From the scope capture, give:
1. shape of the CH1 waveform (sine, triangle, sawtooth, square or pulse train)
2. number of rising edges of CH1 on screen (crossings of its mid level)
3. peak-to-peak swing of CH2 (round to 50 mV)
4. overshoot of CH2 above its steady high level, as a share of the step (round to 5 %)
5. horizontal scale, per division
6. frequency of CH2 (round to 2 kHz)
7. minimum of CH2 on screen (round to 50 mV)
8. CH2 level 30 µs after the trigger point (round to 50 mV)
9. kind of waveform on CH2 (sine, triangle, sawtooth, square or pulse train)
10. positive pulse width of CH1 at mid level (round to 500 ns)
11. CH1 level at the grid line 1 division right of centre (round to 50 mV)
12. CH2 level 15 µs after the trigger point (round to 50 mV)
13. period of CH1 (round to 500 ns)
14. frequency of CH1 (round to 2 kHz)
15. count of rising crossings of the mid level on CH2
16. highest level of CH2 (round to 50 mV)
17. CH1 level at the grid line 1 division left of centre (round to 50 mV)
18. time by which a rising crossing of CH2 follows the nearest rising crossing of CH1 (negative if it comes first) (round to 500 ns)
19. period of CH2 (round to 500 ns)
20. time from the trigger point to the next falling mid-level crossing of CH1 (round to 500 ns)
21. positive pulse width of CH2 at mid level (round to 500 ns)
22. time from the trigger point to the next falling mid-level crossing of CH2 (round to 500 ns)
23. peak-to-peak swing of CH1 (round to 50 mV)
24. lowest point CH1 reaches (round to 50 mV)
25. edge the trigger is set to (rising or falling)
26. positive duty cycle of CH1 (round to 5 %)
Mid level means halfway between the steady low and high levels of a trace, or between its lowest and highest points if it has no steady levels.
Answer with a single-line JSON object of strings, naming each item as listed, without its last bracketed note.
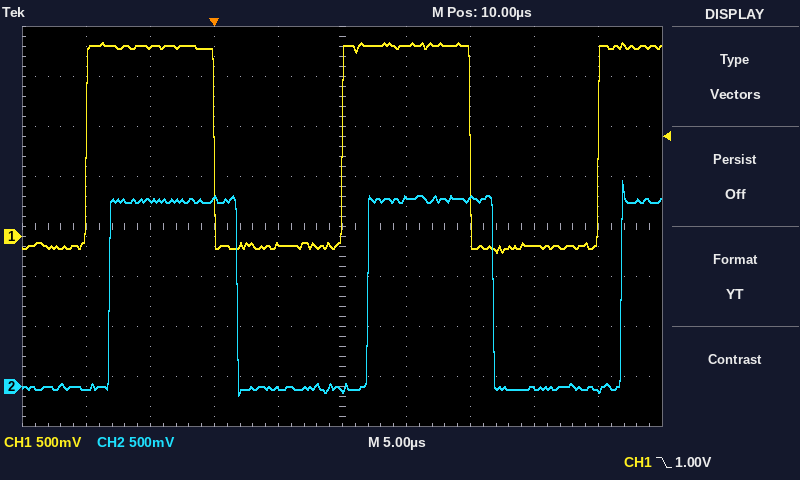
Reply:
{"shape of the CH1 waveform": "square", "number of rising edges of CH1 on screen": "3", "peak-to-peak swing of CH2": "2.15 V", "overshoot of CH2 above its steady high level, as a share of the step": "10 %", "horizontal scale, per division": "5 µs", "frequency of CH2": "50 kHz", "minimum of CH2 on screen": "-100 mV", "CH2 level 30 µs after the trigger point": "-50 mV", "kind of waveform on CH2": "square", "positive pulse width of CH1 at mid level": "10.0 µs", "CH1 level at the grid line 1 division right of centre": "1.90 V", "CH2 level 15 µs after the trigger point": "1.90 V", "period of CH1": "20.0 µs", "frequency of CH1": "50 kHz", "count of rising crossings of the mid level on CH2": "3", "highest level of CH2": "2.05 V", "CH1 level at the grid line 1 division left of centre": "-100 mV", "time by which a rising crossing of CH2 follows the nearest rising crossing of CH1 (negative if it comes first)": "+2.0 µs", "period of CH2": "20.0 µs", "time from the trigger point to the next falling mid-level crossing of CH1": "20.0 µs", "positive pulse width of CH2 at mid level": "10.0 µs", "time from the trigger point to the next falling mid-level crossing of CH2": "2.0 µs", "peak-to-peak swing of CH1": "2.10 V", "lowest point CH1 reaches": "-150 mV", "edge the trigger is set to": "falling", "positive duty cycle of CH1": "50 %"}
